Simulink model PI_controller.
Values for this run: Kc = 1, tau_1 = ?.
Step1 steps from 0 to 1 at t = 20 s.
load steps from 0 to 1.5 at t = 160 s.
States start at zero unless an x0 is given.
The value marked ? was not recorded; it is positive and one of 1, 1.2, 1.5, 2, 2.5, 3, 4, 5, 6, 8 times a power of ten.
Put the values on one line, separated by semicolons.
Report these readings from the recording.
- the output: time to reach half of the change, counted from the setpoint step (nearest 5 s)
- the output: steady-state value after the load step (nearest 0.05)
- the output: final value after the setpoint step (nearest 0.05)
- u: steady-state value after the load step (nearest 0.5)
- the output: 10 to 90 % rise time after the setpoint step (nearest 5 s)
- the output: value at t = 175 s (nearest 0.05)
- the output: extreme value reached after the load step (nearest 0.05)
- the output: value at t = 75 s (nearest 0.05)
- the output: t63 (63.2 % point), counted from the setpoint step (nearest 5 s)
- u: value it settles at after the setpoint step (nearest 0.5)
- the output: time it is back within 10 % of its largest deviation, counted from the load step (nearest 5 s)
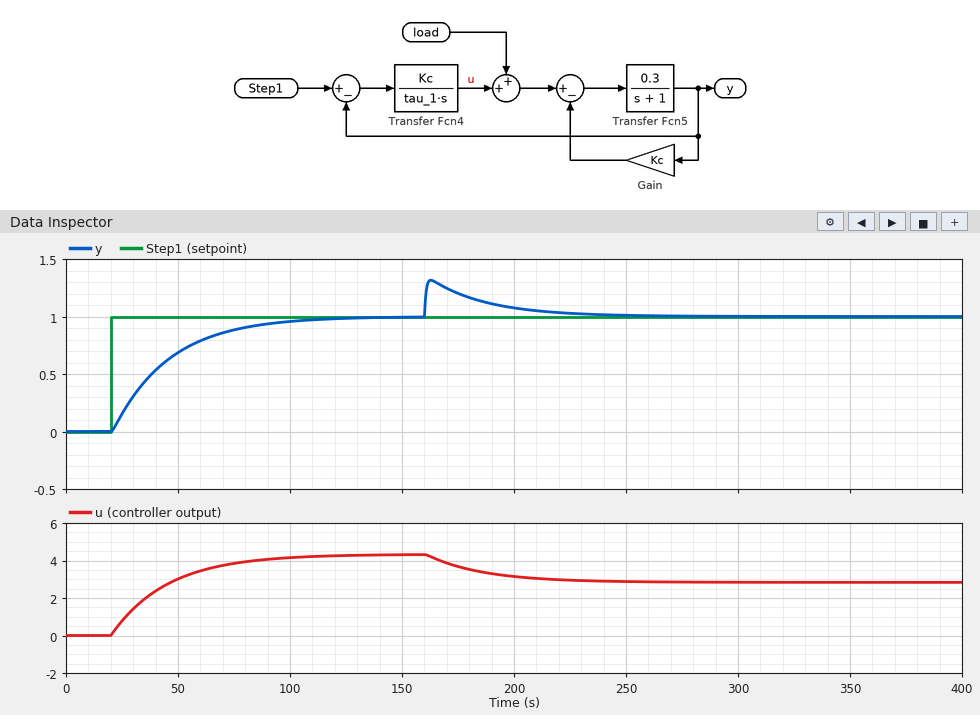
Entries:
20 s; 1.00; 1.00; 3.0; 55 s; 1.20; 1.30; 0.90; 25 s; 4.5; 60 s
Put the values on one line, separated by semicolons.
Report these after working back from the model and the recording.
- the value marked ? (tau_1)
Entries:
6
